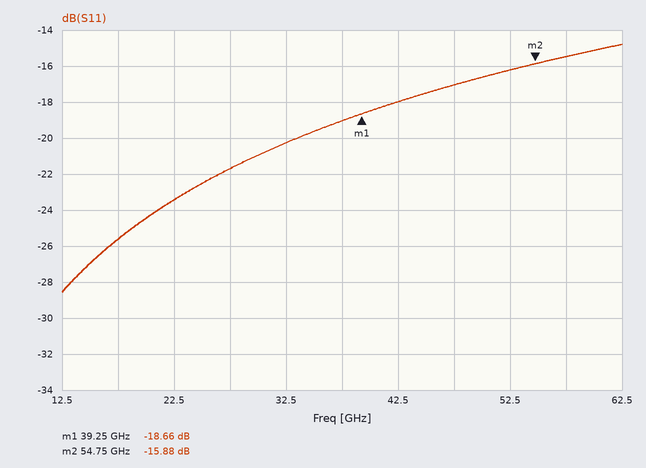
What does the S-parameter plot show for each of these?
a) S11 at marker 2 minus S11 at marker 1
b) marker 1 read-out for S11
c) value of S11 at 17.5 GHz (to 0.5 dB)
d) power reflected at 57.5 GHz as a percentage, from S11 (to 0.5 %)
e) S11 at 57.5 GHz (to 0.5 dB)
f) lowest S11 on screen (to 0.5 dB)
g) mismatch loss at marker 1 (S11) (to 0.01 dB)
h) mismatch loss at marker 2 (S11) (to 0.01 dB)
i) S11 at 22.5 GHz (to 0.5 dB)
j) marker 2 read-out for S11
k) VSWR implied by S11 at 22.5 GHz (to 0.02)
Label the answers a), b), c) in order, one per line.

a) 2.78 dB
b) -18.66 dB
c) -25.5 dB
d) 3.0 %
e) -15.5 dB
f) -28.5 dB
g) 0.06 dB
h) 0.11 dB
i) -23.5 dB
j) -15.88 dB
k) 1.14
